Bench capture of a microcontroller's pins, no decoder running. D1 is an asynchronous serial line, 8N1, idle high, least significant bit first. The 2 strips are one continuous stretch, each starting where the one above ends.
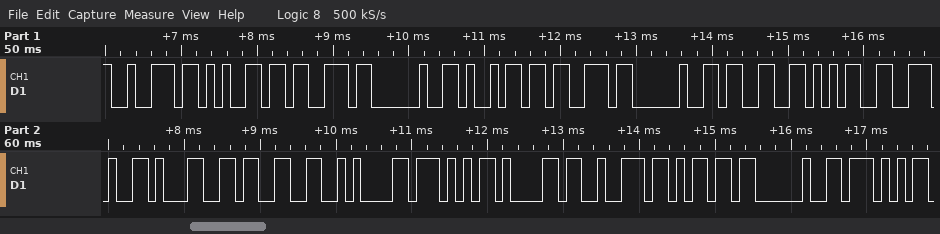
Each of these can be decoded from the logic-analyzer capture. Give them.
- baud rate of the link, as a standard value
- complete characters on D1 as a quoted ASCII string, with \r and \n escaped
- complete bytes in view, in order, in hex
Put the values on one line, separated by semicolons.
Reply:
9600 baud; "res is 35.13\nWarm W"; 0x72 0x65 0x73 0x20 0x69 0x73 0x20 0x33 0x35 0x2E 0x31 0x33 0x0A 0x57 0x61 0x72 0x6D 0x20 0x57
